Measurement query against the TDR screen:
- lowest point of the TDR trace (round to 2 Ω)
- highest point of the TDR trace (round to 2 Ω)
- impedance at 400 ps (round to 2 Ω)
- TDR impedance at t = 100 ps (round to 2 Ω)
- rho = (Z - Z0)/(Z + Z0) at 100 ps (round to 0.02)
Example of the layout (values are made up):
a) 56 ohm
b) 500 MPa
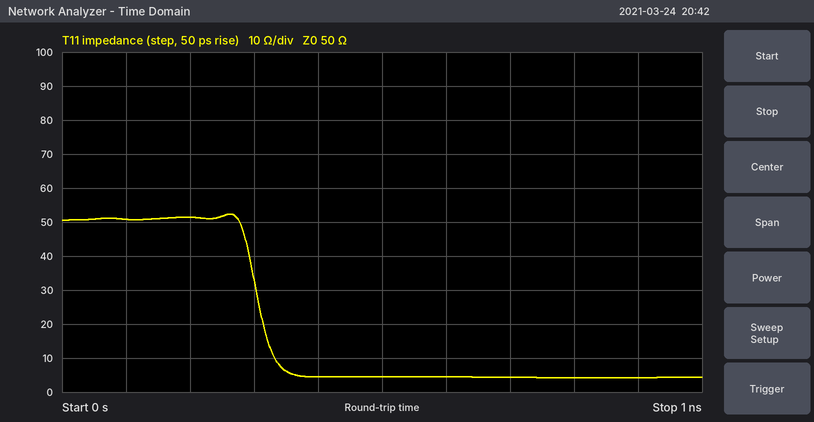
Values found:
a) 4 Ω
b) 52 Ω
c) 4 Ω
d) 50 Ω
e) 0.00
